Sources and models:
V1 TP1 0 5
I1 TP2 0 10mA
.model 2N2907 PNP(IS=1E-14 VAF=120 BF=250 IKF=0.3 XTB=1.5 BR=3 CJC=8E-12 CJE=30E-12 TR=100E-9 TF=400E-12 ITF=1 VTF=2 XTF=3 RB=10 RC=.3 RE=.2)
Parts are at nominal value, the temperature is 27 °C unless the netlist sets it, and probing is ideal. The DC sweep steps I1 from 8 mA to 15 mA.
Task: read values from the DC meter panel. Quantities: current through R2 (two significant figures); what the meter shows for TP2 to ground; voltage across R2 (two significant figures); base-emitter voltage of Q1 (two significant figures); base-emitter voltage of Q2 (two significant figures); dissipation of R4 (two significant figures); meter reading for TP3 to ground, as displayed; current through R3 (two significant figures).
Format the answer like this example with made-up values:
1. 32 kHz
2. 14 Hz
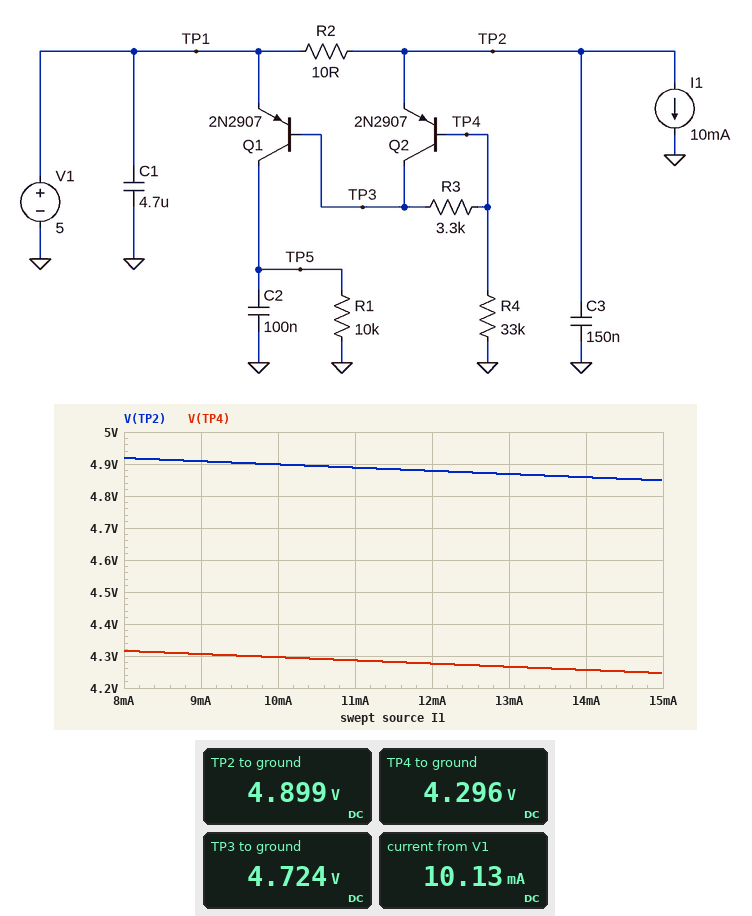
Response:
1. 10 mA
2. 4.899 V
3. 100 mV
4. -280 mV
5. -600 mV
6. 560 µW
7. 4.724 V
8. 130 µA
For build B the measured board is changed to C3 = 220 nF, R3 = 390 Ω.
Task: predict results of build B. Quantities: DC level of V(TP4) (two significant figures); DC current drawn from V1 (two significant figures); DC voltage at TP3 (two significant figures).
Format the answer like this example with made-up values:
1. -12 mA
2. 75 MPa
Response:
1. 4.3 V
2. 11 mA
3. 4.4 V
